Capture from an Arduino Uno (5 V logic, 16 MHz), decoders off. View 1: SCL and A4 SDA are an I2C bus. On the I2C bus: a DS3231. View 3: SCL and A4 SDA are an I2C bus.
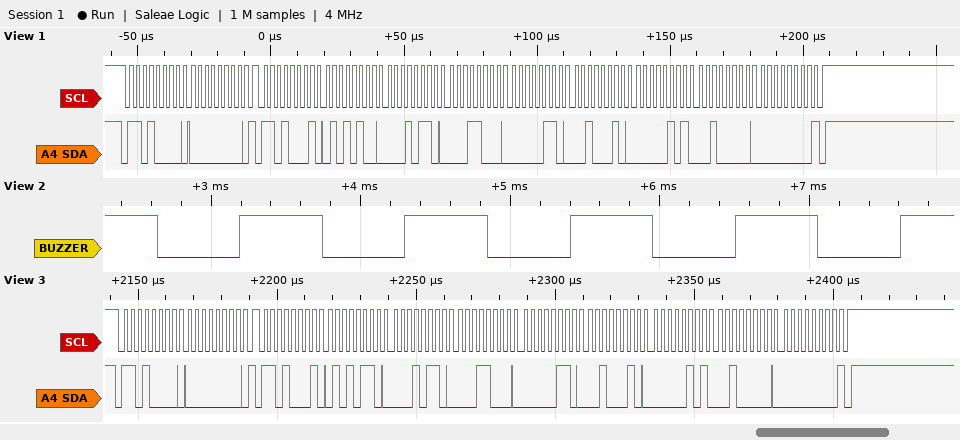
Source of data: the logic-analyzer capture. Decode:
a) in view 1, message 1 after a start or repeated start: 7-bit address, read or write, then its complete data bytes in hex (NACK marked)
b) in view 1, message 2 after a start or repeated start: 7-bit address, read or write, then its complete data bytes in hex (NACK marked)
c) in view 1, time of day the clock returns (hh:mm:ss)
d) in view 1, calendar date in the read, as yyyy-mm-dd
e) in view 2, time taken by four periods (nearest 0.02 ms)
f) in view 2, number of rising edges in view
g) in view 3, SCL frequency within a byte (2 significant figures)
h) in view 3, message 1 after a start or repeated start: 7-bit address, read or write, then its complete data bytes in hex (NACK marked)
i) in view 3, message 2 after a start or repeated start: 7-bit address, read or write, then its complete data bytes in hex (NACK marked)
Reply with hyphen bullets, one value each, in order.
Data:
- 0x68 write: 00
- 0x68 read: 54 16 18 06 22 05 20 00 NACK
- 18:16:54
- 2020-05-22
- 4.42 ms
- 5
- 400 kHz
- 0x68 write: 00
- 0x68 read: 56 16 18 06 22 05 20 00 NACK
